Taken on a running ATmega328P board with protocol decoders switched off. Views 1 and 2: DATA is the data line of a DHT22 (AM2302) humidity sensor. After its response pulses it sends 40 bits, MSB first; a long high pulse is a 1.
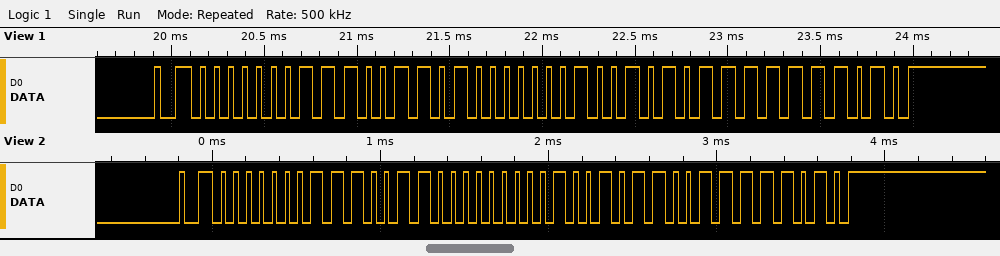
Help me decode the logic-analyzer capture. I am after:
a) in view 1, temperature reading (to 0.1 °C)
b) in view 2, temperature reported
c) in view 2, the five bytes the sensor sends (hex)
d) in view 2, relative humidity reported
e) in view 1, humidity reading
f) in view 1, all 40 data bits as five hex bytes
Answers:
29.9 °C
30.0 °C
01 CC 01 2C FA
46.0 %
46.1 %
01 CD 01 2B FA
